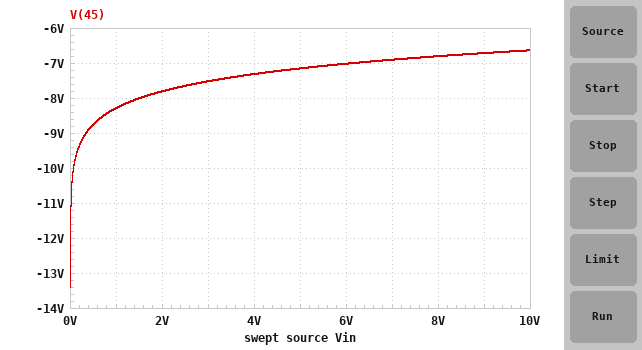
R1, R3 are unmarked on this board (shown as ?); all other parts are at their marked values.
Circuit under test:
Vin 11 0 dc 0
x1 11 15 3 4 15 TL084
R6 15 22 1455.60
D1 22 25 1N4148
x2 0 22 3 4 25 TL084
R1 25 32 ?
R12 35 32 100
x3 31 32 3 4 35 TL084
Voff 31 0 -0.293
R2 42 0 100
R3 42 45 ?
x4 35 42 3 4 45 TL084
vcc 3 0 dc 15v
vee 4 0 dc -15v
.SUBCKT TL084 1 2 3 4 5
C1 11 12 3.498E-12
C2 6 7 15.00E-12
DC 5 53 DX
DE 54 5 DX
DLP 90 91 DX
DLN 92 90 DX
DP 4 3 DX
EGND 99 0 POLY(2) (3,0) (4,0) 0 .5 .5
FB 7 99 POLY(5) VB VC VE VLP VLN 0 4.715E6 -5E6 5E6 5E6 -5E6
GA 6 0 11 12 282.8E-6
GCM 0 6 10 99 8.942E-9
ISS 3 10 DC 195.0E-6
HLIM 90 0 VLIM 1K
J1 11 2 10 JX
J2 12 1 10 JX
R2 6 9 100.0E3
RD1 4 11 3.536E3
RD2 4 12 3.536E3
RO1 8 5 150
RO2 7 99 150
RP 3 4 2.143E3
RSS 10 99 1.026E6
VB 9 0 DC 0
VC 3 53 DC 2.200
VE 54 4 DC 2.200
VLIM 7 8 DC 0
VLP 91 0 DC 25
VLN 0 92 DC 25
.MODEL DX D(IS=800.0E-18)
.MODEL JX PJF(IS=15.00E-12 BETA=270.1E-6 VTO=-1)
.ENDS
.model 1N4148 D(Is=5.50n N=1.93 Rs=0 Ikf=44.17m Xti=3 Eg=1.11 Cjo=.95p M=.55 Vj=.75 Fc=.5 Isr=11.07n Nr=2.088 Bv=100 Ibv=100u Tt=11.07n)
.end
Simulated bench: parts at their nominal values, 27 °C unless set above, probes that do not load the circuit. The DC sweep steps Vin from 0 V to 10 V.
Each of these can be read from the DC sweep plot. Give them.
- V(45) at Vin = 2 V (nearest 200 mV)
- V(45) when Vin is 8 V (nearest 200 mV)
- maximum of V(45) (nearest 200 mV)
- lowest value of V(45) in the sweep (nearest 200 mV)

-7.8 V
-6.8 V
-6.6 V
-13.4 V
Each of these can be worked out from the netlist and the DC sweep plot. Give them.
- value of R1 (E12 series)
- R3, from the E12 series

330 Ω
3.9 kΩ
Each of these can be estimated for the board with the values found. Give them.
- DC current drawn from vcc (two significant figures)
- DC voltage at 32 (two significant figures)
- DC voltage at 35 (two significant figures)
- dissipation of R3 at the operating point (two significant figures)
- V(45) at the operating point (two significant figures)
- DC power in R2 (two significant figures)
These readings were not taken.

57 mA
-290 mV
-380 mV
44 mW
-13 V
1.1 mW
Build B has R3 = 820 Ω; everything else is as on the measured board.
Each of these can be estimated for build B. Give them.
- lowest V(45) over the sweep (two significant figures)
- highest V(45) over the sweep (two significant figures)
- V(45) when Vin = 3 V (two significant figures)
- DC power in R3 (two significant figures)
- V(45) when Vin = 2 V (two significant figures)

-3.5 V
-1.5 V
-1.7 V
12 mW
-1.8 V
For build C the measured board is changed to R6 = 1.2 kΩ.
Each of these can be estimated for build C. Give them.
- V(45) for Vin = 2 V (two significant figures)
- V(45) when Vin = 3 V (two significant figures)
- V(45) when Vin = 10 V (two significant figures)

-7.7 V
-7.4 V
-6.5 V
